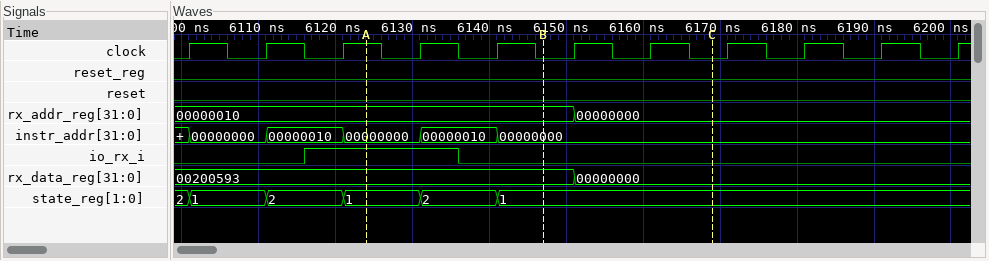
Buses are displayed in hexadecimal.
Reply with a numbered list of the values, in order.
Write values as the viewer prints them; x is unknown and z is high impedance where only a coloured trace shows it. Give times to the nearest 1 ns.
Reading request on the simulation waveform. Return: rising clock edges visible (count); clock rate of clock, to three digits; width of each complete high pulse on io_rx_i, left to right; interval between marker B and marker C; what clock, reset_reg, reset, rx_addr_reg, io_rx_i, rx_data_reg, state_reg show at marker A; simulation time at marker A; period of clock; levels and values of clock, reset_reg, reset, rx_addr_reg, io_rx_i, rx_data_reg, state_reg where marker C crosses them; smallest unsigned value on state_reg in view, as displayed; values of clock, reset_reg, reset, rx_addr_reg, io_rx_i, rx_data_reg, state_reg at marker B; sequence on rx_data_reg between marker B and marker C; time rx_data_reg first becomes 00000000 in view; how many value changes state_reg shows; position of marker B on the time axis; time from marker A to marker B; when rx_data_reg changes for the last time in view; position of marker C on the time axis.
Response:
1. 11
2. 100 MHz
3. 20 ns
4. 22 ns
5. clock=1, reset_reg=0, reset=0, rx_addr_reg=00000010, io_rx_i=1, rx_data_reg=00200593, state_reg=1
6. 6124 ns
7. 10 ns
8. clock=0, reset_reg=0, reset=0, rx_addr_reg=00000000, io_rx_i=0, rx_data_reg=00000000, state_reg=1
9. 1
10. clock=0, reset_reg=0, reset=0, rx_addr_reg=00000010, io_rx_i=0, rx_data_reg=00200593, state_reg=1
11. 00200593, 00000000
12. 6151 ns
13. 5
14. 6147 ns
15. 23 ns
16. 6151 ns
17. 6169 ns
